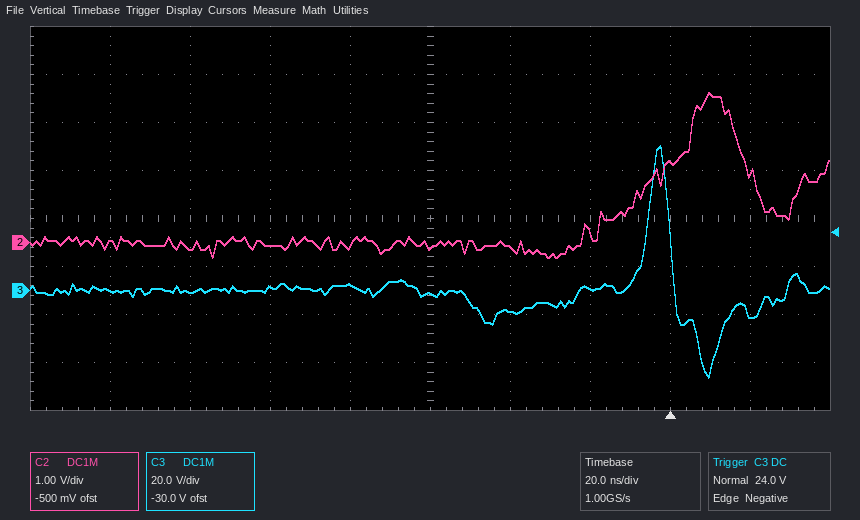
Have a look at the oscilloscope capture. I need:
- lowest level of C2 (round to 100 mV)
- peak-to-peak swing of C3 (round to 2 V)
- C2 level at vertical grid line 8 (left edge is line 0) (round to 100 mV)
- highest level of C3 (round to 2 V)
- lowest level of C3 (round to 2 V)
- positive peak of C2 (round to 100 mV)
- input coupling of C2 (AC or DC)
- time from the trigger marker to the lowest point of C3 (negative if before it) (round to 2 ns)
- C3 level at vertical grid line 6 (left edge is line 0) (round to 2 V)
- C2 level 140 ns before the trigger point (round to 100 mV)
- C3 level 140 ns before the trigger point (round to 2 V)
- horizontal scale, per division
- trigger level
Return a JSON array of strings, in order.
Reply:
["-300 mV", "96 V", "1.7 V", "60 V", "-36 V", "3.1 V", "DC", "+10 ns", "-8 V", "0.0 V", "0 V", "20 ns", "24.0 V"]
